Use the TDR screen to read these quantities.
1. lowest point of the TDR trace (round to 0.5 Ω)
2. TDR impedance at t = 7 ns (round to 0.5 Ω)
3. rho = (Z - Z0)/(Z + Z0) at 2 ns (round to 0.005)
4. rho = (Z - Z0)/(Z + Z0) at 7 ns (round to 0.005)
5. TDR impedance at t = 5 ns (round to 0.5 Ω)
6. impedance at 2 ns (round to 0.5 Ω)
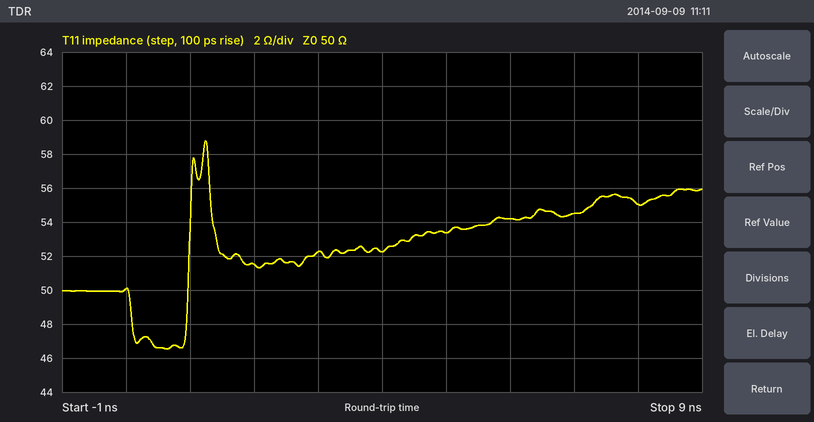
46.5 Ω
54.5 Ω
+0.015
+0.045
53.5 Ω
51.5 Ω
